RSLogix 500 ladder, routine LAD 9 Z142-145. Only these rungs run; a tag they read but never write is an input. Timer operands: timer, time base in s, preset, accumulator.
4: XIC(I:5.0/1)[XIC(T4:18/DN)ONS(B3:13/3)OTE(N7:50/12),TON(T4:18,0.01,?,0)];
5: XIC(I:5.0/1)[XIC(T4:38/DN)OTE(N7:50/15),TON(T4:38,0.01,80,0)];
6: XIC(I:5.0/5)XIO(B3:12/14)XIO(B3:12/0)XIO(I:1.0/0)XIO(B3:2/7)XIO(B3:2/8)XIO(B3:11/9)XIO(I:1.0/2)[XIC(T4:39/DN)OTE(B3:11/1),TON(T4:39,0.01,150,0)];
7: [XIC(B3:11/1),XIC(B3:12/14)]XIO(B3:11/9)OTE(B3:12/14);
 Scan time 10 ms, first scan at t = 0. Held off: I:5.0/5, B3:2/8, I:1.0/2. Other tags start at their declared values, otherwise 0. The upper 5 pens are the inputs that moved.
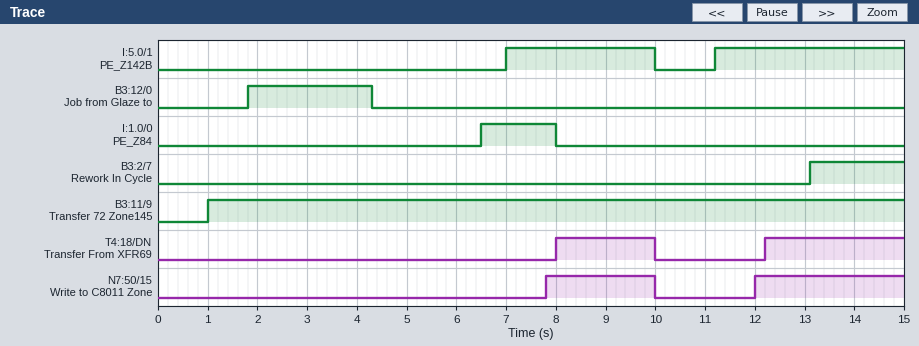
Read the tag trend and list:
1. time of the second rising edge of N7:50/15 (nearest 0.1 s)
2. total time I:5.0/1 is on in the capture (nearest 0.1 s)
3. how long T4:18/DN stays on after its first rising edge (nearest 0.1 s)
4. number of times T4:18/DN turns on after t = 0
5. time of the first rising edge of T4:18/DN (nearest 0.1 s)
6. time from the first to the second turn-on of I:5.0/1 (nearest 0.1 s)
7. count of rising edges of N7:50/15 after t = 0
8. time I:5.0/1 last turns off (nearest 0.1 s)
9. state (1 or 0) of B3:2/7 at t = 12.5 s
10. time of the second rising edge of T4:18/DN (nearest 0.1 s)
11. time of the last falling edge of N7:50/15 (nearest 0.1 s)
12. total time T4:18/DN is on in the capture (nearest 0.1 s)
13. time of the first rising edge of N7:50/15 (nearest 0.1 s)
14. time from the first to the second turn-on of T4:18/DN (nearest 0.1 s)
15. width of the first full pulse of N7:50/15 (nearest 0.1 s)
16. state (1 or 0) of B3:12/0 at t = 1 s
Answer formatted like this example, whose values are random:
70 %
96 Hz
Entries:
12.0 s
6.8 s
2.0 s
2
8.0 s
4.2 s
2
10.0 s
0
12.2 s
10.0 s
4.8 s
7.8 s
4.2 s
2.2 s
0
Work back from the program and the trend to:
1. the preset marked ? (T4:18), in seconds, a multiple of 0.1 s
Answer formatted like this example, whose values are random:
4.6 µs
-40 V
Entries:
1.0 s
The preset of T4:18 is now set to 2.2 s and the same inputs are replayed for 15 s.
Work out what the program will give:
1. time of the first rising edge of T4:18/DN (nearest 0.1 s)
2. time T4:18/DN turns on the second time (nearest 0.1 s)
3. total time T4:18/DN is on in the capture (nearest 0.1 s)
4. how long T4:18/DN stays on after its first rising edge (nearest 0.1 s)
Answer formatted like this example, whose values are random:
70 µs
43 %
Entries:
9.2 s
13.4 s
2.4 s
0.8 s
